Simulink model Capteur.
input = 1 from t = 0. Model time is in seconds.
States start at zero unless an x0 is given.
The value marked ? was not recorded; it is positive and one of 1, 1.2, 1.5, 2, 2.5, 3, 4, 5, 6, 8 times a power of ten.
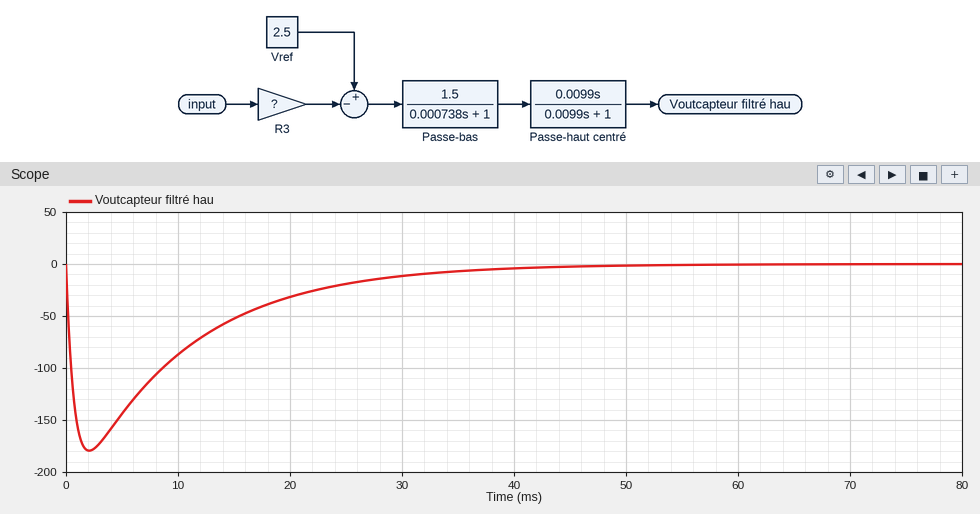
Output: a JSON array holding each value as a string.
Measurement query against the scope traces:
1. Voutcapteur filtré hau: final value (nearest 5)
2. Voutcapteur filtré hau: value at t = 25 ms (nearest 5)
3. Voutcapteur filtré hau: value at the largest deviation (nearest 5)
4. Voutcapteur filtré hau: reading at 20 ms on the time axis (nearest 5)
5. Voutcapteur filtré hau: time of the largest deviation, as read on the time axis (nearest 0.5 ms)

["0", "-20", "-180", "-30", "2.0 ms"]
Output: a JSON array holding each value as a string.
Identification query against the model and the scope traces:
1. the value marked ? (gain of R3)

["150"]
